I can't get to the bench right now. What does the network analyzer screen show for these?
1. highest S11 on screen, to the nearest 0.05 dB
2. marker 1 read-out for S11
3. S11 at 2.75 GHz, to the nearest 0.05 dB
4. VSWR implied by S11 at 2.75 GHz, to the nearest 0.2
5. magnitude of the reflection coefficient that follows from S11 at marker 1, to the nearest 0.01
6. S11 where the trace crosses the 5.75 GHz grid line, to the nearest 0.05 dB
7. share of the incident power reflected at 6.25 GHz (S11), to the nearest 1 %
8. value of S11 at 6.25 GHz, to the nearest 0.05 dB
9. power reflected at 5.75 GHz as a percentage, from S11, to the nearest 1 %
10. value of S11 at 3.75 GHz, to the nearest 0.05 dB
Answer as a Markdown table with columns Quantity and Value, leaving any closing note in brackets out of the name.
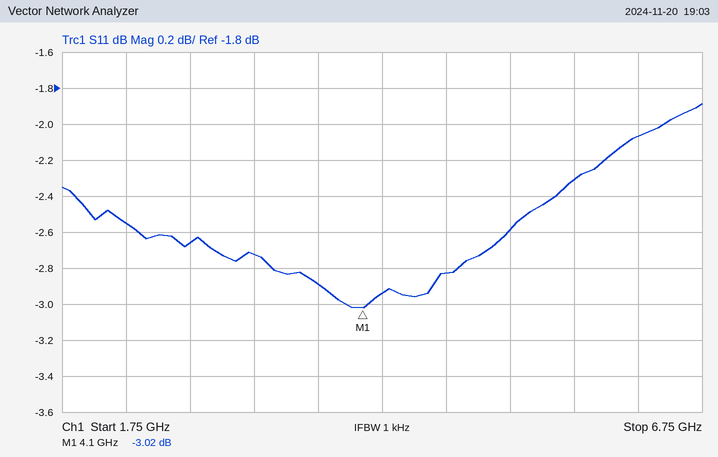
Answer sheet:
| Quantity | Value |
|---|---|
| highest S11 on screen, to the nearest 0.05 dB | -1.90 dB |
| marker 1 read-out for S11 | -3.02 dB |
| S11 at 2.75 GHz, to the nearest 0.05 dB | -2.65 dB |
| VSWR implied by S11 at 2.75 GHz, to the nearest 0.2 | 6.6 |
| magnitude of the reflection coefficient that follows from S11 at marker 1, to the nearest 0.01 | 0.71 |
| S11 where the trace crosses the 5.75 GHz grid line, to the nearest 0.05 dB | -2.30 dB |
| share of the incident power reflected at 6.25 GHz (S11), to the nearest 1 % | 62 % |
| value of S11 at 6.25 GHz, to the nearest 0.05 dB | -2.05 dB |
| power reflected at 5.75 GHz as a percentage, from S11, to the nearest 1 % | 59 % |
| value of S11 at 3.75 GHz, to the nearest 0.05 dB | -2.90 dB |
